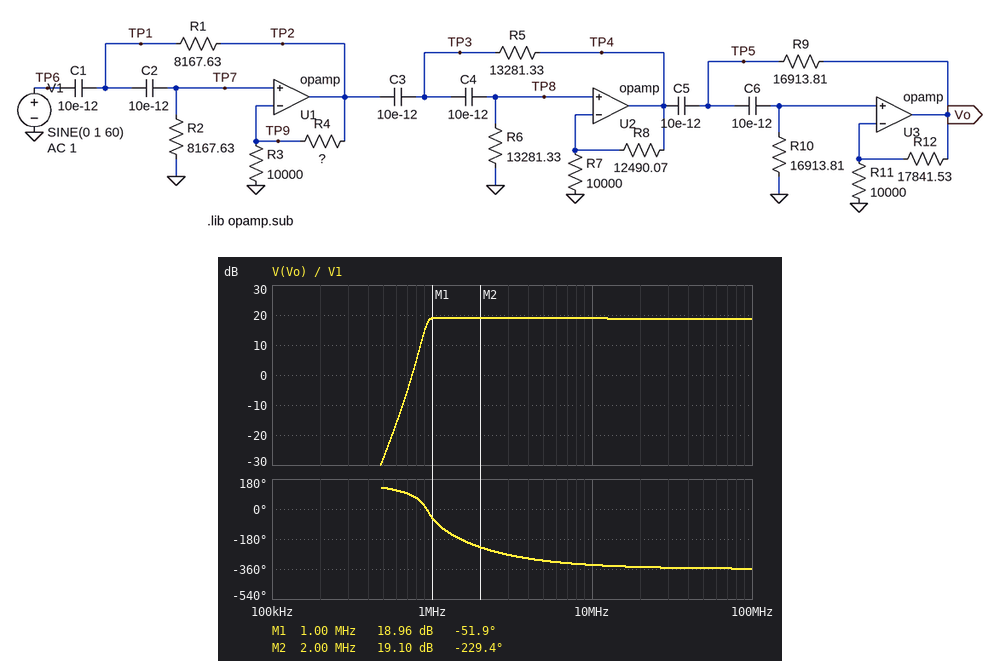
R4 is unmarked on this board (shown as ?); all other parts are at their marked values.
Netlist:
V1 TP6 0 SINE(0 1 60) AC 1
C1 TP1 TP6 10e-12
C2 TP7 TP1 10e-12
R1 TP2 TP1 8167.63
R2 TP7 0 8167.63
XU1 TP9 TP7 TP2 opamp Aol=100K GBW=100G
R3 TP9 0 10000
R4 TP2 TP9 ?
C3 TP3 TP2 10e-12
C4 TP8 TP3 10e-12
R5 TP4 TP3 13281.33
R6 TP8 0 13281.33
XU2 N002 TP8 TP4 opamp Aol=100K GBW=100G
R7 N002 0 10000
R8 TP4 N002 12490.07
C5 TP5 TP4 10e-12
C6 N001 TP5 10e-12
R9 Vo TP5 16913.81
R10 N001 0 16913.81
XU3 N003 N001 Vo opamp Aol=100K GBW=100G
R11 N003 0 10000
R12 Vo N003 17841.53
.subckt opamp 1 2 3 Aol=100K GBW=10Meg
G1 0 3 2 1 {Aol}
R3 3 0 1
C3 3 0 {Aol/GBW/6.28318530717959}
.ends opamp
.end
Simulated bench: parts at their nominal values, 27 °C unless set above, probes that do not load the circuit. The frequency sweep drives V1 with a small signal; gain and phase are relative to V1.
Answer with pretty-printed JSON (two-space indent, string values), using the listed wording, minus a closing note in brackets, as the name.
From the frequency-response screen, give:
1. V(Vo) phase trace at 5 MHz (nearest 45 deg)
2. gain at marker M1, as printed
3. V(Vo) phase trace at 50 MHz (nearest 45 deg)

{
  "V(Vo) phase trace at 5 MHz": "-315 deg",
  "gain at marker M1, as printed": "18.96 dB",
  "V(Vo) phase trace at 50 MHz": "-360 deg"
}
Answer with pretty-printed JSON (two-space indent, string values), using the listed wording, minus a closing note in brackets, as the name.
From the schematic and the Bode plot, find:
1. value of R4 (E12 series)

{
  "value of R4": "3.9 kΩ"
}
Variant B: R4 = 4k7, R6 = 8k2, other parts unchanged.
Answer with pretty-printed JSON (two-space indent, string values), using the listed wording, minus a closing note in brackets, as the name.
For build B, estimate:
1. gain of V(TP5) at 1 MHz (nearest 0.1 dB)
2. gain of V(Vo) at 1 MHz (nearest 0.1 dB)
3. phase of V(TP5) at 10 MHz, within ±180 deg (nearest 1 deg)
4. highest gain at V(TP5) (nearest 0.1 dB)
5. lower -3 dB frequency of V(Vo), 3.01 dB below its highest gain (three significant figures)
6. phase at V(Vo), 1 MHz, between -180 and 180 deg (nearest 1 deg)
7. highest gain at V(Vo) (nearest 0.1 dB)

{
  "gain of V(TP5) at 1 MHz": "4.8 dB",
  "gain of V(Vo) at 1 MHz": "11.0 dB",
  "phase of V(TP5) at 10 MHz, within ±180 deg": "27 deg",
  "highest gain at V(TP5)": "10.4 dB",
  "lower -3 dB frequency of V(Vo), 3.01 dB below its highest gain": "2.10 MHz",
  "phase at V(Vo), 1 MHz, between -180 and 180 deg": "-47 deg",
  "highest gain at V(Vo)": "19.3 dB"
}
